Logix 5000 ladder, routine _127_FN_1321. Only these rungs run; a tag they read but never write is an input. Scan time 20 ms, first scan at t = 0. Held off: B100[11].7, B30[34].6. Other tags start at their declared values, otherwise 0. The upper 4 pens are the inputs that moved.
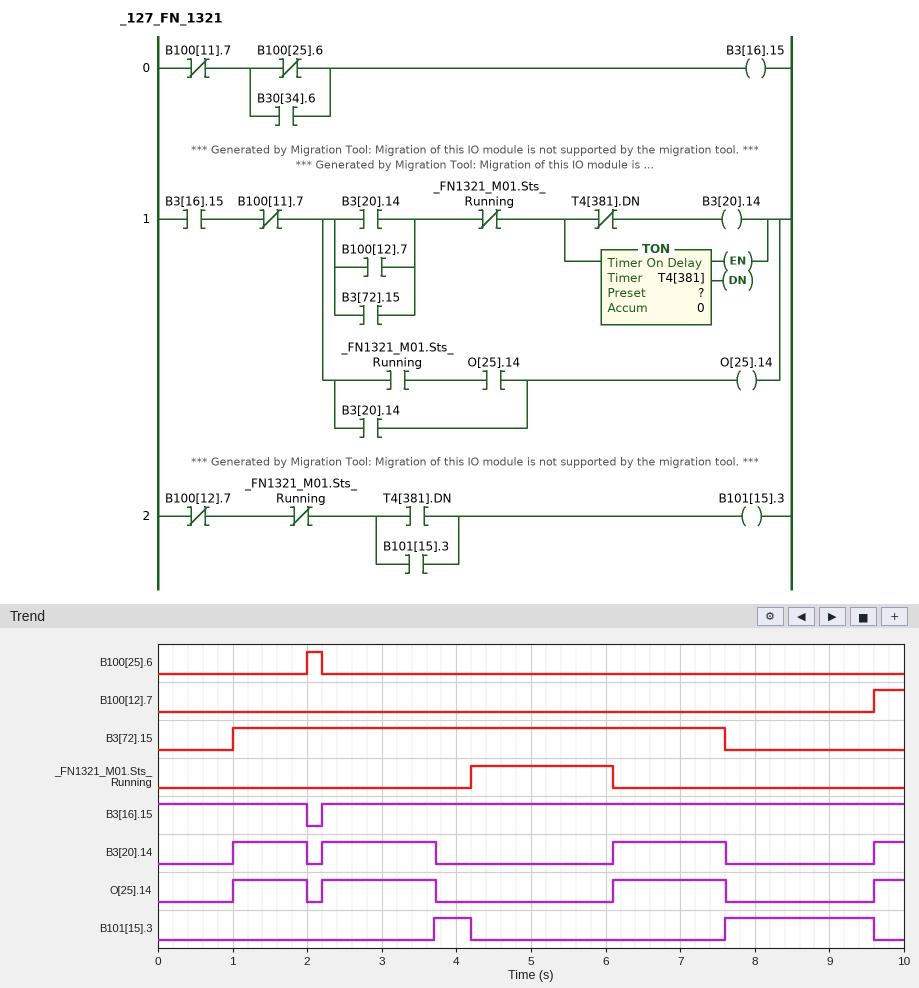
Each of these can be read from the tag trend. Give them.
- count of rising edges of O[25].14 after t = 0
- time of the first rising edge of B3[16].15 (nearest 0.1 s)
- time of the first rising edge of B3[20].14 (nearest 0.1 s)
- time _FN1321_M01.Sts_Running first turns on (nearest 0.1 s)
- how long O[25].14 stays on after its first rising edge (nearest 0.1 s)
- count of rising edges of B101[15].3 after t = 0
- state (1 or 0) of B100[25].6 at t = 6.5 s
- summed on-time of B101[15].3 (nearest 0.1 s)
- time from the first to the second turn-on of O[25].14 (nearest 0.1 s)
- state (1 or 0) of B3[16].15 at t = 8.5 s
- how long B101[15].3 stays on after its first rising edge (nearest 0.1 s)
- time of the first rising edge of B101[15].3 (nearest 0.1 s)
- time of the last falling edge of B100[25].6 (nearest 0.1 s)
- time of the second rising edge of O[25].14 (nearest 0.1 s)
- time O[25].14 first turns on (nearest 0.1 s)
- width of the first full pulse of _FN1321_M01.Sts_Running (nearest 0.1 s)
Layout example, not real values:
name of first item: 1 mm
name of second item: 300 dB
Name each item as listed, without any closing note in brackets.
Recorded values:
count of rising edges of O[25].14 after t = 0: 4
time of the first rising edge of B3[16].15: 2.2 s
time of the first rising edge of B3[20].14: 1.0 s
time _FN1321_M01.Sts_Running first turns on: 4.2 s
how long O[25].14 stays on after its first rising edge: 1.0 s
count of rising edges of B101[15].3 after t = 0: 2
state (1 or 0) of B100[25].6 at t = 6.5 s: 0
summed on-time of B101[15].3: 2.5 s
time from the first to the second turn-on of O[25].14: 1.2 s
state (1 or 0) of B3[16].15 at t = 8.5 s: 1
how long B101[15].3 stays on after its first rising edge: 0.5 s
time of the first rising edge of B101[15].3: 3.7 s
time of the last falling edge of B100[25].6: 2.2 s
time of the second rising edge of O[25].14: 2.2 s
time O[25].14 first turns on: 1.0 s
width of the first full pulse of _FN1321_M01.Sts_Running: 1.9 s
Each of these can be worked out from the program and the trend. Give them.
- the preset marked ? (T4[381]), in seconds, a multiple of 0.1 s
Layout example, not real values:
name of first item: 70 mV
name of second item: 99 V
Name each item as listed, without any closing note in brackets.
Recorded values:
the preset marked ? (T4[381]), in seconds, a multiple of 0.1 s: 1.5 s
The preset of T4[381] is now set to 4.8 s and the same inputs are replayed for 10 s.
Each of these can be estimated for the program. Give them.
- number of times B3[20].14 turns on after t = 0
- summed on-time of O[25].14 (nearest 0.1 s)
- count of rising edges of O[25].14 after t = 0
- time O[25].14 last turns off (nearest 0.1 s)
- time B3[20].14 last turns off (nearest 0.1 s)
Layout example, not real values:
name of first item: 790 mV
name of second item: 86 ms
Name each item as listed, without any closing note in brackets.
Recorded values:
number of times B3[20].14 turns on after t = 0: 3
summed on-time of O[25].14: 8.8 s
count of rising edges of O[25].14 after t = 0: 2
time O[25].14 last turns off: 2.0 s
time B3[20].14 last turns off: 4.2 s
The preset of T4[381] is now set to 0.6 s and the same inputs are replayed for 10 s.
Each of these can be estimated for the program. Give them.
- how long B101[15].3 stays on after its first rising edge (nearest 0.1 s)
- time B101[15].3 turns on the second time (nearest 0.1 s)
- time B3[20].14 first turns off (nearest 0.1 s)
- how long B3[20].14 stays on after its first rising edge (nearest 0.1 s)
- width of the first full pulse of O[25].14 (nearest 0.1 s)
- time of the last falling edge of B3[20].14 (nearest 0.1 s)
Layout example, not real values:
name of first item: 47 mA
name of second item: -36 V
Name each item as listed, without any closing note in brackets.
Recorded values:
how long B101[15].3 stays on after its first rising edge: 2.6 s
time B101[15].3 turns on the second time: 6.7 s
time B3[20].14 first turns off: 1.6 s
how long B3[20].14 stays on after its first rising edge: 0.6 s
width of the first full pulse of O[25].14: 0.6 s
time of the last falling edge of B3[20].14: 6.7 s
